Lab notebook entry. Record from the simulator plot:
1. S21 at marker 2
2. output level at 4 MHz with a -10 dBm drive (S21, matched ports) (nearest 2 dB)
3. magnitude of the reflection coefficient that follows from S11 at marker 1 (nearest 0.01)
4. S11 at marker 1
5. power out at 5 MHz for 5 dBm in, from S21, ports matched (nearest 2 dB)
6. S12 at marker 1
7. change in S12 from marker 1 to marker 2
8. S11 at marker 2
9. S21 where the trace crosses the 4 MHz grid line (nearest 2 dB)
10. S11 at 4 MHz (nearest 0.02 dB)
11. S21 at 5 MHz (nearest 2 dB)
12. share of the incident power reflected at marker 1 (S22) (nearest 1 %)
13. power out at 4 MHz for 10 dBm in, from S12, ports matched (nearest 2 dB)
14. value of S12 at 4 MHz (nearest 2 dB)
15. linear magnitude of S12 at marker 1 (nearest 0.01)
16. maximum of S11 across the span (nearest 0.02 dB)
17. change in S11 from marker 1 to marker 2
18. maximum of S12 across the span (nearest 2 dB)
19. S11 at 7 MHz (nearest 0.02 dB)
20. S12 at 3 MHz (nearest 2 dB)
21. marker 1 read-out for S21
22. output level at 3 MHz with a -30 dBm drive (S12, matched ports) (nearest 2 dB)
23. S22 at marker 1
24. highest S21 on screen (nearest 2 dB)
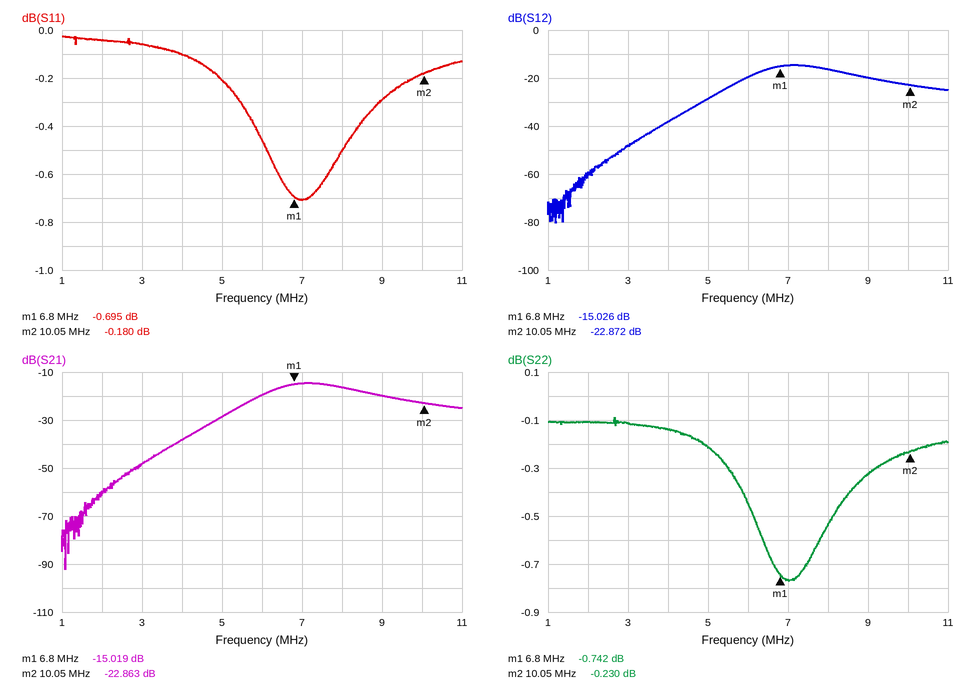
-22.863 dB
-48 dBm
0.92
-0.695 dB
-24 dBm
-15.026 dB
-7.846 dB
-0.180 dB
-38 dB
-0.10 dB
-28 dB
84 %
-28 dBm
-38 dB
0.18
-0.02 dB
0.515 dB
-14 dB
-0.70 dB
-48 dB
-15.019 dB
-78 dBm
-0.742 dB
-14 dB
